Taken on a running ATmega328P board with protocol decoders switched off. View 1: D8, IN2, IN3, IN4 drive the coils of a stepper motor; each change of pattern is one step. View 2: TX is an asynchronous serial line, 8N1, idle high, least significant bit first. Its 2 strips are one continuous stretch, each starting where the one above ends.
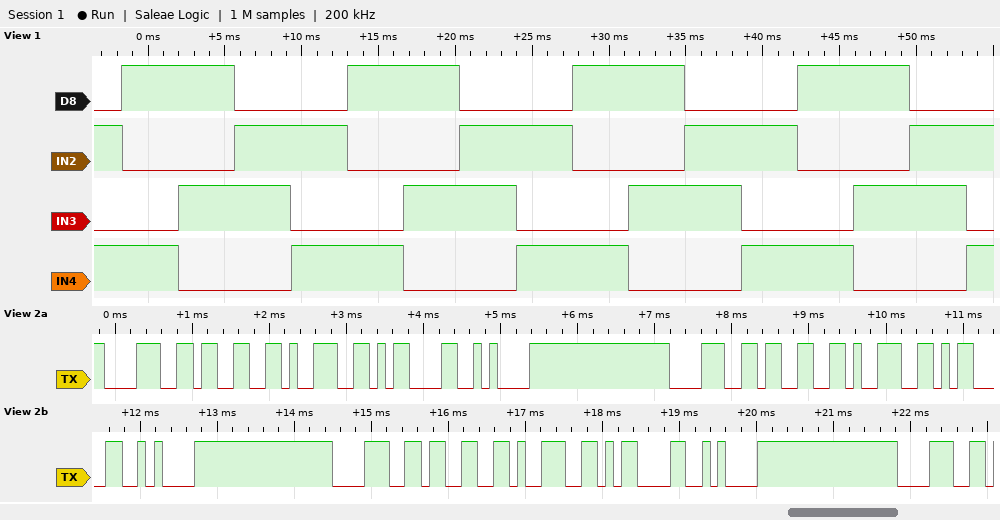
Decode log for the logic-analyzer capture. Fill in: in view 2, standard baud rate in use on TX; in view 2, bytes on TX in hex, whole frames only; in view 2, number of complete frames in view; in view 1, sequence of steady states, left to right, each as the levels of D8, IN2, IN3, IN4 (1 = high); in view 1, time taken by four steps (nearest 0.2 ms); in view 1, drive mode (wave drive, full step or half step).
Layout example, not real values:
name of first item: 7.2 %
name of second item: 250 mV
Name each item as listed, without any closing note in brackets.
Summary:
in view 2, standard baud rate in use on TX: 9600 baud
in view 2, bytes on TX in hex, whole frames only: 0x38 0x33 0x39 0x0D 0x0A 0x38 0x33 0x39 0x0D 0x0A 0x38 0x33 0x39 0x0D 0x0A 0x38
in view 2, number of complete frames in view: 16
in view 1, sequence of steady states, left to right, each as the levels of D8, IN2, IN3, IN4: 0101 1001 1010 0110 0101 1001 1010 0110 0101 1001 1010 0110 0101 1001 1010 0110 0101
in view 1, time taken by four steps: 14.6 ms
in view 1, drive mode: full step
